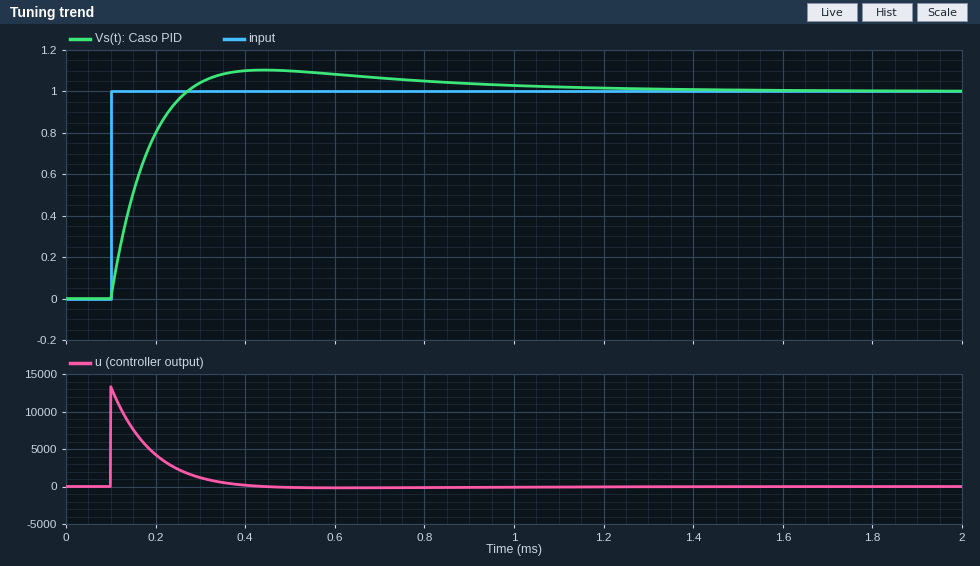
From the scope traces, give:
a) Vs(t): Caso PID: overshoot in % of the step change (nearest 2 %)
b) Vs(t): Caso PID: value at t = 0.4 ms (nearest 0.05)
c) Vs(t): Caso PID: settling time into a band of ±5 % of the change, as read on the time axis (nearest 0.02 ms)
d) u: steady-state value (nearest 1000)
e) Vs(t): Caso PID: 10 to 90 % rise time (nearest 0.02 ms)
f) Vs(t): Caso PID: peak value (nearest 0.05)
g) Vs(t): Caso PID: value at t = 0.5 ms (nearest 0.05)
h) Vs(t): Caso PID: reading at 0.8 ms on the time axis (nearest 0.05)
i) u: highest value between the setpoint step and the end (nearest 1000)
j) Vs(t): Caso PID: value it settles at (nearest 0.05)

10 %
1.10
0.80 ms
0
0.12 ms
1.10
1.10
1.05
13000
1.00
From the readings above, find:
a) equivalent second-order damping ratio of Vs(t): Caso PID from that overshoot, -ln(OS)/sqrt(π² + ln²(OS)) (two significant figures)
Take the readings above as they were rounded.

0.59
